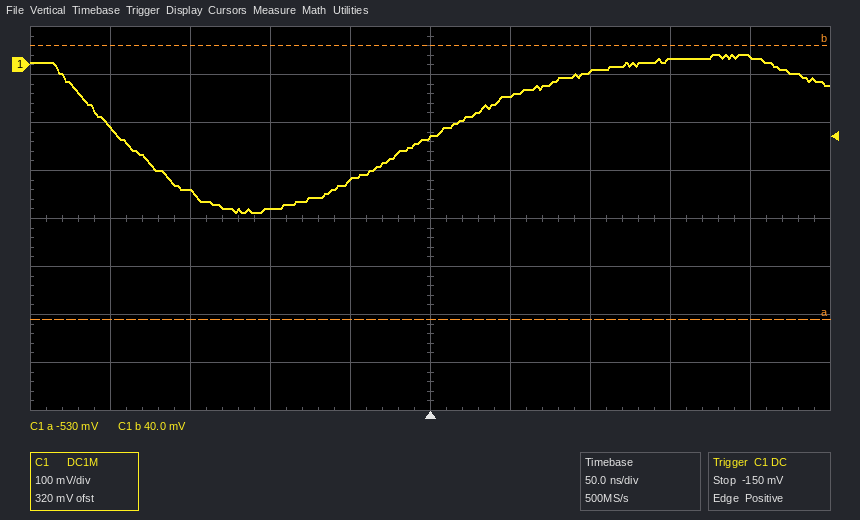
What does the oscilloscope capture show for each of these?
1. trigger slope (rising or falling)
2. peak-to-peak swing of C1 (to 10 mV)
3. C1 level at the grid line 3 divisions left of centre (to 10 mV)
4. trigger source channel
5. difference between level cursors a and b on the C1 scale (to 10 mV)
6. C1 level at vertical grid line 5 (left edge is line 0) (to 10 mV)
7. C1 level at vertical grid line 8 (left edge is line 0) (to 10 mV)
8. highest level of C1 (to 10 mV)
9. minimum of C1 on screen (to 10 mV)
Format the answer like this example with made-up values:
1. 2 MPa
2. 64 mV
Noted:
1. rising
2. 330 mV
3. -260 mV
4. C1
5. 570 mV
6. -150 mV
7. 10 mV
8. 20 mV
9. -310 mV
